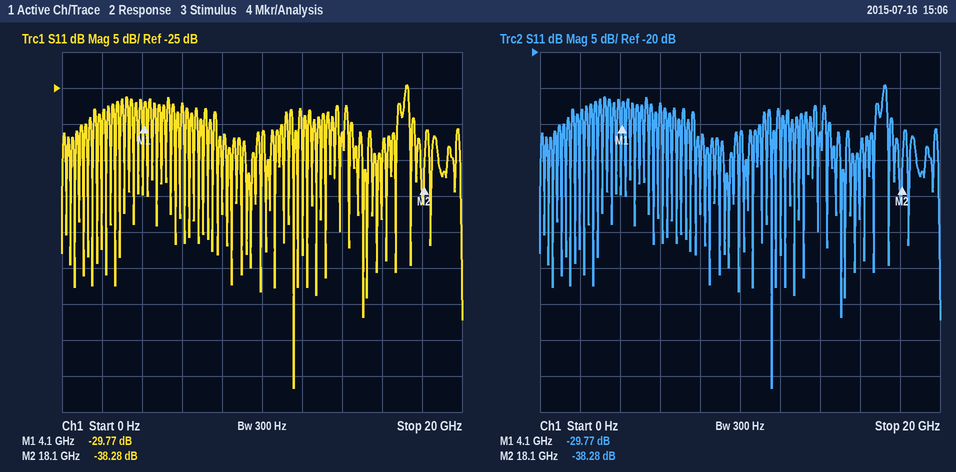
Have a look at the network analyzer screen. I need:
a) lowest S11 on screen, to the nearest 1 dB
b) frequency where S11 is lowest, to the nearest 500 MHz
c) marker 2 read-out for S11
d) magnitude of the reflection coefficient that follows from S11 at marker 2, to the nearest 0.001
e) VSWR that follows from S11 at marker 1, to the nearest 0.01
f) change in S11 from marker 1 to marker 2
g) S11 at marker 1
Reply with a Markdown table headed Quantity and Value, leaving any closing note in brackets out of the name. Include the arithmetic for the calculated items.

| Quantity | Value |
|---|---|
| lowest S11 on screen, to the nearest 1 dB | -67 dB |
| frequency where S11 is lowest, to the nearest 500 MHz | 11.5 GHz |
| marker 2 read-out for S11 | -38.28 dB |
| magnitude of the reflection coefficient that follows from S11 at marker 2, to the nearest 0.001 | 10^(-38.28/20) ≈ 0.012 |
| VSWR that follows from S11 at marker 1, to the nearest 0.01 | (1 + 0.0325)/(1 − 0.0325) ≈ 1.07 |
| change in S11 from marker 1 to marker 2 | -38.28 − (-29.77) = -8.51 dB |
| S11 at marker 1 | -29.77 dB |
